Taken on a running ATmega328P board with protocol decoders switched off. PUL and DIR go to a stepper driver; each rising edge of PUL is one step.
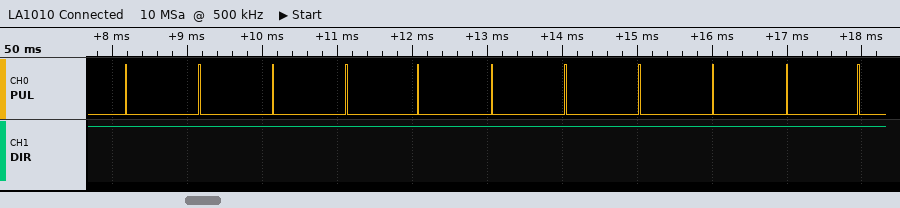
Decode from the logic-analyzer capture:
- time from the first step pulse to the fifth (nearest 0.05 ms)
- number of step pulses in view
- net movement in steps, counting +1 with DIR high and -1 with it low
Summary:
3.90 ms
11
+11
